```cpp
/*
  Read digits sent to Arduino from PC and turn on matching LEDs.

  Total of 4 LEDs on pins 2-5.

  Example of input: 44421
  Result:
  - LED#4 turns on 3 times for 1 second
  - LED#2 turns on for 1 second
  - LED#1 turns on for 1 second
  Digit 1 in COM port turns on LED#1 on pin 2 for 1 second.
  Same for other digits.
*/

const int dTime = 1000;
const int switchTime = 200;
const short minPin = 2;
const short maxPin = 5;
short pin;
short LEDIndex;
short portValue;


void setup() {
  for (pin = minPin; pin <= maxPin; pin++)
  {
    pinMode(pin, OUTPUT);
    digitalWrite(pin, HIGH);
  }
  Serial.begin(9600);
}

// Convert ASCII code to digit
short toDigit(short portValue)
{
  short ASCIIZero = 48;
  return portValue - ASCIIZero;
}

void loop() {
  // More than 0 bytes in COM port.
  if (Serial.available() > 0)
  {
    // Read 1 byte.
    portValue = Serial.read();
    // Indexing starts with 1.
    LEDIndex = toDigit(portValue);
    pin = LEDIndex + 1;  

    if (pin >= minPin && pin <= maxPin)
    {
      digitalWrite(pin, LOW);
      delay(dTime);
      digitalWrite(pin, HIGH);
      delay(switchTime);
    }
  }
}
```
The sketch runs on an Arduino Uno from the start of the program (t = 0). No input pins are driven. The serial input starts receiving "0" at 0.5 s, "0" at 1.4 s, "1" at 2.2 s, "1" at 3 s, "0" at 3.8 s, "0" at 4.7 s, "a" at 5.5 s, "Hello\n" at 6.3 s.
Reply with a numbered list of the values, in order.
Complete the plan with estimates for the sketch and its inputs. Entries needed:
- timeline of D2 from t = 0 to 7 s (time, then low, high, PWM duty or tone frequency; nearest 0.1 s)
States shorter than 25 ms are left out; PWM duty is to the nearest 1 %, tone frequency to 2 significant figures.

1. 0 s high; 2.2 s low; 3.2 s high; 3.4 s low; 4.4 s high
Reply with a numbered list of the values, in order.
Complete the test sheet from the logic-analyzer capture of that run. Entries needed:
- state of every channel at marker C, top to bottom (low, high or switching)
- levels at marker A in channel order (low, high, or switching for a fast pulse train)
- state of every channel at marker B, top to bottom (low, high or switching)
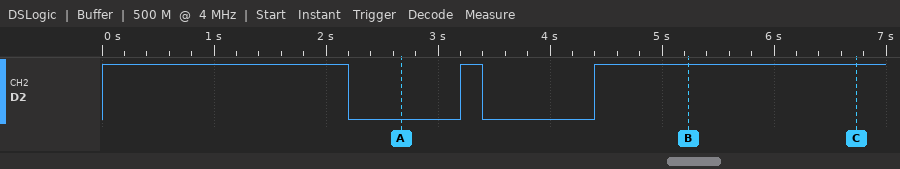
1. D2 high
2. D2 low
3. D2 high
